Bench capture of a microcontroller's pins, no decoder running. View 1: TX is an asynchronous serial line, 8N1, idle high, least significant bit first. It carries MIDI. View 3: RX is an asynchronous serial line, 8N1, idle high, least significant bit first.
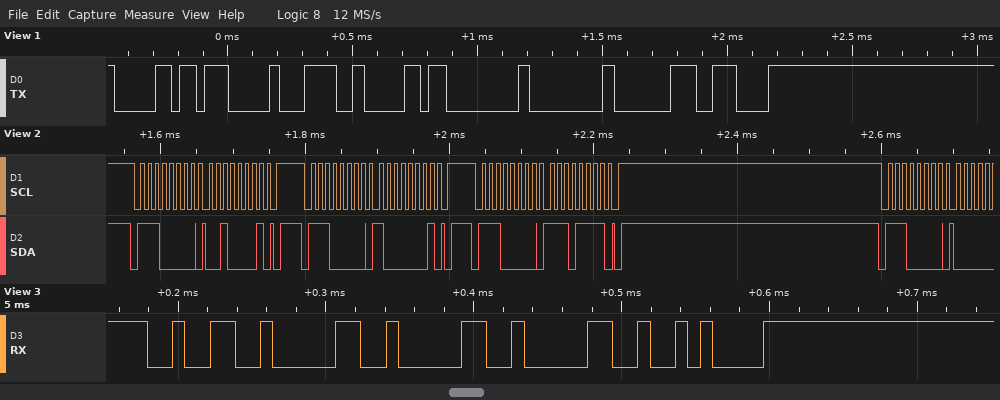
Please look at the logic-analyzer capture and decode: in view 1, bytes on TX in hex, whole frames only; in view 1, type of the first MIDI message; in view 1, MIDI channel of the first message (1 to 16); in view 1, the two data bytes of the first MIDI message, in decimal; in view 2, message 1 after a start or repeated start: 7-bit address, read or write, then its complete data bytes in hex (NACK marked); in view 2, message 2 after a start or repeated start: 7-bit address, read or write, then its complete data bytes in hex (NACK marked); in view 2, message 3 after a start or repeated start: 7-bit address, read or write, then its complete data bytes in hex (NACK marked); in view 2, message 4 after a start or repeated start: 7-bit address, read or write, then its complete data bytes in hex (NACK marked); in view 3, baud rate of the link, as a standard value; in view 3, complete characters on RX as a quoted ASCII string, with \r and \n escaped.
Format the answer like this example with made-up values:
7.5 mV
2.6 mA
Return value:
B0 07 3C B0 00 00 C0 0E
Control Change
1
7, 60
0x70 write: 21
0x70 write: 81
0x70 write: EF
0x70 write
115200 baud
"2000\n"
